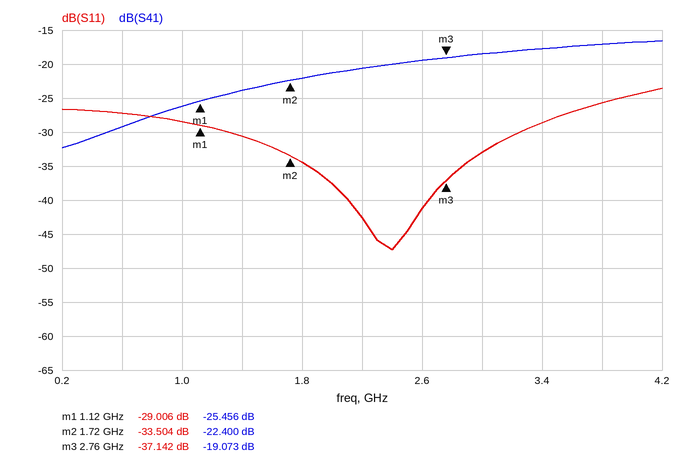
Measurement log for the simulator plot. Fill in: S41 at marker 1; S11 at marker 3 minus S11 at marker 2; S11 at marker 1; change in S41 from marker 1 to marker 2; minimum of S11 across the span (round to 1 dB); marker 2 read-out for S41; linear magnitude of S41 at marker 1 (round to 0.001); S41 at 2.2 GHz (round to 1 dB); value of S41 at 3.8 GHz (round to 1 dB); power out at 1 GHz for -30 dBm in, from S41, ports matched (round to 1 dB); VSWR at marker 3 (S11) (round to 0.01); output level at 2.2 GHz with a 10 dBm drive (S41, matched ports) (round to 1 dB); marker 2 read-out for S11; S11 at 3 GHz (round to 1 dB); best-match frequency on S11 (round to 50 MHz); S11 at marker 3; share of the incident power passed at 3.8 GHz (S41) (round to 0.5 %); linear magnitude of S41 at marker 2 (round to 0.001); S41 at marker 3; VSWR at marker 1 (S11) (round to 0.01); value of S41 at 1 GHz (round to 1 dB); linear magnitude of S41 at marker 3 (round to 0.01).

-25.456 dB
-3.638 dB
-29.006 dB
3.056 dB
-47 dB
-22.400 dB
0.053
-21 dB
-17 dB
-56 dBm
1.03
-11 dBm
-33.504 dB
-33 dB
2.40 GHz
-37.142 dB
2.0 %
0.076
-19.073 dB
1.07
-26 dB
0.11
